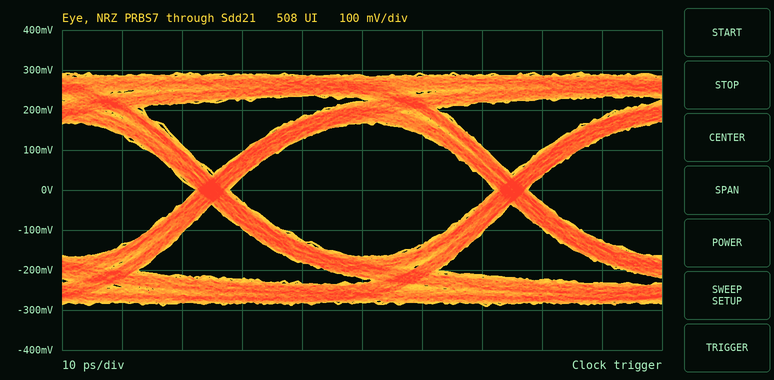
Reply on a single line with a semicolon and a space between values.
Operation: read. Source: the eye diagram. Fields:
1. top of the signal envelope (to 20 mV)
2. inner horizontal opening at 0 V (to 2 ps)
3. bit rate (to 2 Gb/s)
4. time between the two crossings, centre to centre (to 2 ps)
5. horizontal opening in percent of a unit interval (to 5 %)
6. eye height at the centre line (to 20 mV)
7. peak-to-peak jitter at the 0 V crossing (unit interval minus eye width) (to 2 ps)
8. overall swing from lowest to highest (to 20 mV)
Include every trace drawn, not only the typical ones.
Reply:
300 mV; 44 ps; 20 Gb/s; 50 ps; 90 %; 340 mV; 6 ps; 580 mV
